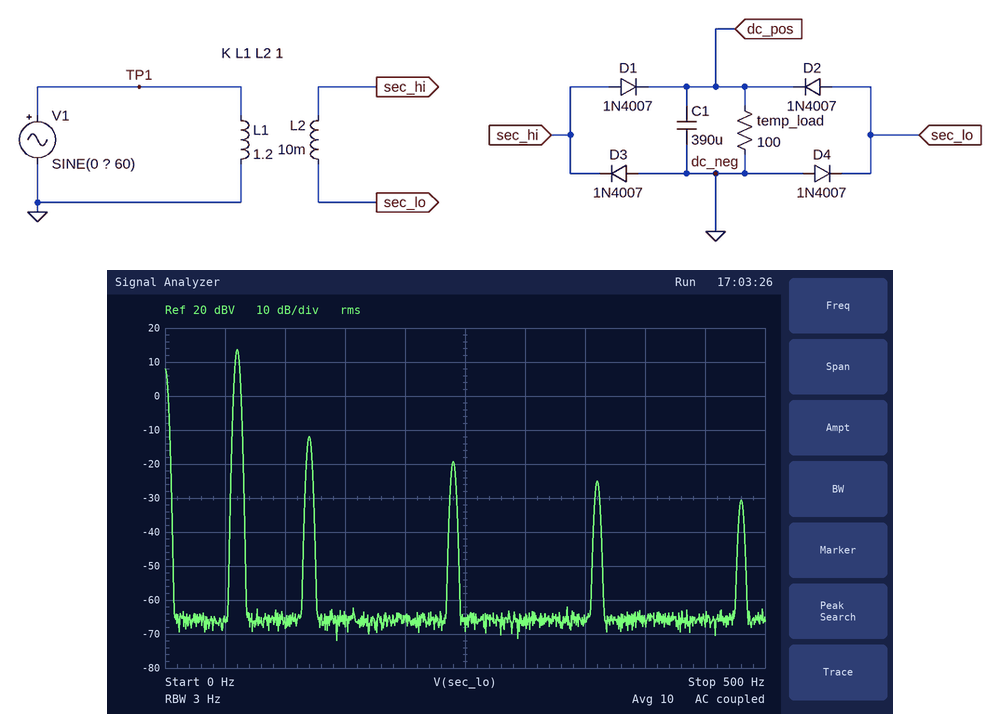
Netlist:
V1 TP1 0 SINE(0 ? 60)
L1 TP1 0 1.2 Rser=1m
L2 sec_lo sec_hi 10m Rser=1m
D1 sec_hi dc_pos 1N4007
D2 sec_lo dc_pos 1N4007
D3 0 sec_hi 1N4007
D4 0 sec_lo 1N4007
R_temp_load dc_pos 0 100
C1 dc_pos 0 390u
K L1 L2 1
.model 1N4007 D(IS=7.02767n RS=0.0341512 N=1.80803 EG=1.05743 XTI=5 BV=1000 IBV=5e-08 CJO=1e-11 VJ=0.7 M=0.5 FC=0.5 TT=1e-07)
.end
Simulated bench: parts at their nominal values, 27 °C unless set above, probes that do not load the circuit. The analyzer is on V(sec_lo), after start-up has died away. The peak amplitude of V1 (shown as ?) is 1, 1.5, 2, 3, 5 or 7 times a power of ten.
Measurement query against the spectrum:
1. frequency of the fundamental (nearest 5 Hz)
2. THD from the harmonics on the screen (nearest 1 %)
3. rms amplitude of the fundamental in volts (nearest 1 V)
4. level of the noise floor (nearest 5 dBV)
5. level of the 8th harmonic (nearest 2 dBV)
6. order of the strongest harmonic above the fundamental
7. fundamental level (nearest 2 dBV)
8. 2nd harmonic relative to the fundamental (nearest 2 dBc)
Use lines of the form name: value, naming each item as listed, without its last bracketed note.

frequency of the fundamental: 60 Hz
THD from the harmonics on the screen: 6 %
rms amplitude of the fundamental in volts: 5 V
level of the noise floor: -65 dBV
level of the 8th harmonic: -30 dBV
order of the strongest harmonic above the fundamental: 2
fundamental level: 14 dBV
2nd harmonic relative to the fundamental: -26 dBc
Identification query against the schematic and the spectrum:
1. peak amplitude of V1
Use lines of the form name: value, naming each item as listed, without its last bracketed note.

peak amplitude of V1: 150 V
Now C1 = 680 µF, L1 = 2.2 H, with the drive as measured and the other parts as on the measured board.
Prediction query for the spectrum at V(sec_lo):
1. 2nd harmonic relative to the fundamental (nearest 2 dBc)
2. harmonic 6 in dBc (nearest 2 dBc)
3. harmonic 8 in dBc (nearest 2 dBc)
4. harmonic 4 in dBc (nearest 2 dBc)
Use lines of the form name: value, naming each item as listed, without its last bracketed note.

2nd harmonic relative to the fundamental: -30 dBc
harmonic 6 in dBc: -42 dBc
harmonic 8 in dBc: -48 dBc
harmonic 4 in dBc: -38 dBc
